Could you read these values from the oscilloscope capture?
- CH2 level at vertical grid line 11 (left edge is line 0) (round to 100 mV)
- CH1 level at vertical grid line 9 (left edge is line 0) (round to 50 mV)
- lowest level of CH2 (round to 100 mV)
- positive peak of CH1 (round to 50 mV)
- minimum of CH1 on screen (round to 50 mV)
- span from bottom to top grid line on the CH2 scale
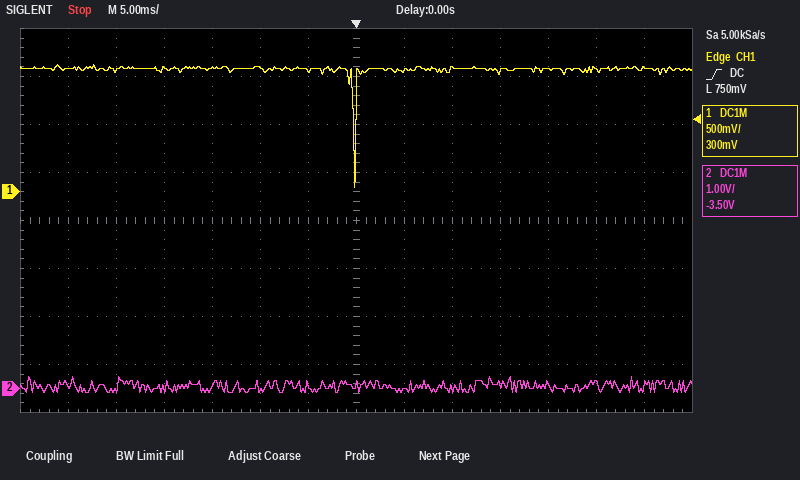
100 mV
1.30 V
-100 mV
1.30 V
50 mV
8 V
